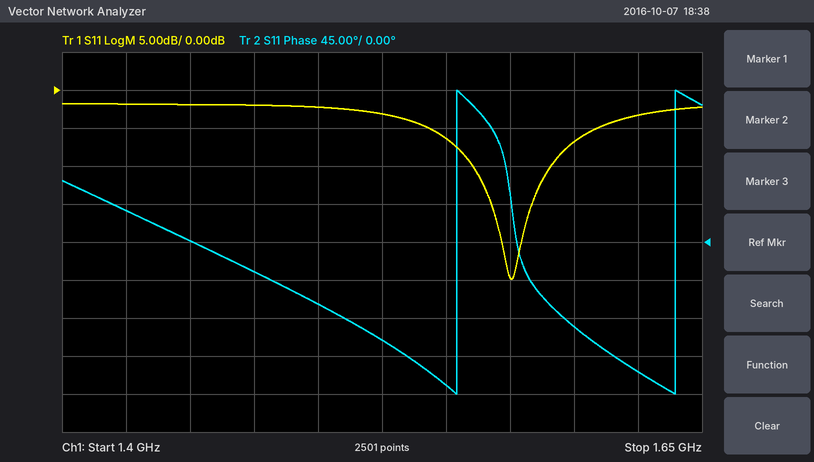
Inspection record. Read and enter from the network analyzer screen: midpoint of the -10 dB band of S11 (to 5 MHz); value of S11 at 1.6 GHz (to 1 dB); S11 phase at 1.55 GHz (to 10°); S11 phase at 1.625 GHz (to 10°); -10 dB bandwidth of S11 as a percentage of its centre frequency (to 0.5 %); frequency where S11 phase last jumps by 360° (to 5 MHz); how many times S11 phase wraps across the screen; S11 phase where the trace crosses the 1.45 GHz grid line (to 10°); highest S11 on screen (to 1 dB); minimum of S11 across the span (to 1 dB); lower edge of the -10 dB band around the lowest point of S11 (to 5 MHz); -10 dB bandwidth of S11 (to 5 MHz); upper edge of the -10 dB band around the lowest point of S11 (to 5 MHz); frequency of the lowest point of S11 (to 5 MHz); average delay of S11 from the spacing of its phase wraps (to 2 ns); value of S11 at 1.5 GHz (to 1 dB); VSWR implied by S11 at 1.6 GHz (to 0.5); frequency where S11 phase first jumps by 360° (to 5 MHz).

1.575 GHz
-7 dB
-170°
-150°
2.0 %
1.640 GHz
2
0°
-2 dB
-25 dB
1.560 GHz
30 MHz
1.590 GHz
1.575 GHz
12 ns
-2 dB
2.5
1.555 GHz
